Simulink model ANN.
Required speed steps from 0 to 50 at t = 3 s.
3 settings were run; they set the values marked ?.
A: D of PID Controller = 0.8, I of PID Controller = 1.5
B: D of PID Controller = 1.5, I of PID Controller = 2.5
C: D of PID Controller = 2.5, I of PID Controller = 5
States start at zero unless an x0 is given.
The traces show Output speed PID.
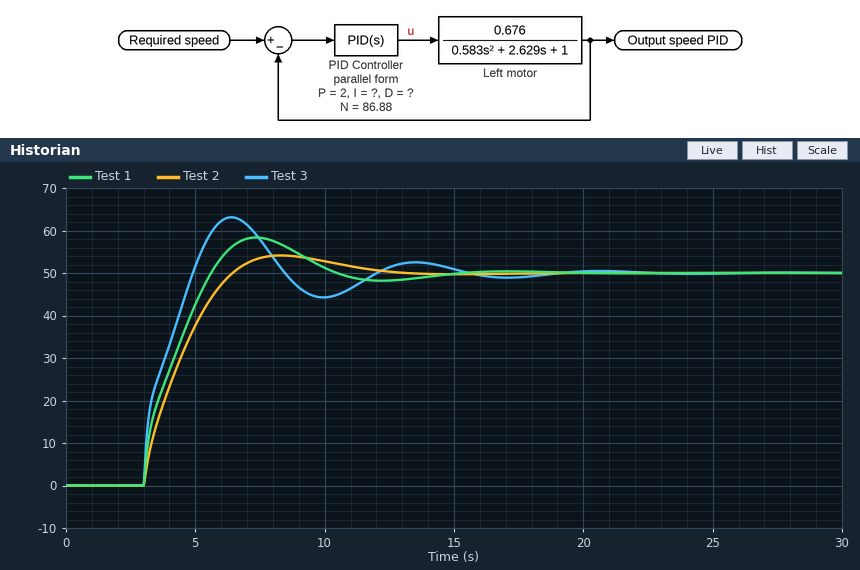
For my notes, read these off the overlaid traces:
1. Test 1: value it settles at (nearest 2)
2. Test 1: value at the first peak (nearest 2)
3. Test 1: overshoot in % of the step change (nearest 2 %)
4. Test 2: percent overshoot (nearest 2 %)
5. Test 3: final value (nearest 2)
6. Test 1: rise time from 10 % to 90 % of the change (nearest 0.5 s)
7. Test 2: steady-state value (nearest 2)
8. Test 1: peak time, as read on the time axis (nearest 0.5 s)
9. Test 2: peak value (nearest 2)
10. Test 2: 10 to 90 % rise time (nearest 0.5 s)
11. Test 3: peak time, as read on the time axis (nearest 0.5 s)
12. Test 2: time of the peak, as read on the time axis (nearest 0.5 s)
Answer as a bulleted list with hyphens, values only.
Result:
- 50
- 58
- 16 %
- 8 %
- 50
- 2.0 s
- 50
- 7.5 s
- 54
- 2.5 s
- 6.5 s
- 8.5 s
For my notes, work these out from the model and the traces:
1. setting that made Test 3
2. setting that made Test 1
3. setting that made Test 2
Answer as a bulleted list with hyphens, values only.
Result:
- C
- B
- A
